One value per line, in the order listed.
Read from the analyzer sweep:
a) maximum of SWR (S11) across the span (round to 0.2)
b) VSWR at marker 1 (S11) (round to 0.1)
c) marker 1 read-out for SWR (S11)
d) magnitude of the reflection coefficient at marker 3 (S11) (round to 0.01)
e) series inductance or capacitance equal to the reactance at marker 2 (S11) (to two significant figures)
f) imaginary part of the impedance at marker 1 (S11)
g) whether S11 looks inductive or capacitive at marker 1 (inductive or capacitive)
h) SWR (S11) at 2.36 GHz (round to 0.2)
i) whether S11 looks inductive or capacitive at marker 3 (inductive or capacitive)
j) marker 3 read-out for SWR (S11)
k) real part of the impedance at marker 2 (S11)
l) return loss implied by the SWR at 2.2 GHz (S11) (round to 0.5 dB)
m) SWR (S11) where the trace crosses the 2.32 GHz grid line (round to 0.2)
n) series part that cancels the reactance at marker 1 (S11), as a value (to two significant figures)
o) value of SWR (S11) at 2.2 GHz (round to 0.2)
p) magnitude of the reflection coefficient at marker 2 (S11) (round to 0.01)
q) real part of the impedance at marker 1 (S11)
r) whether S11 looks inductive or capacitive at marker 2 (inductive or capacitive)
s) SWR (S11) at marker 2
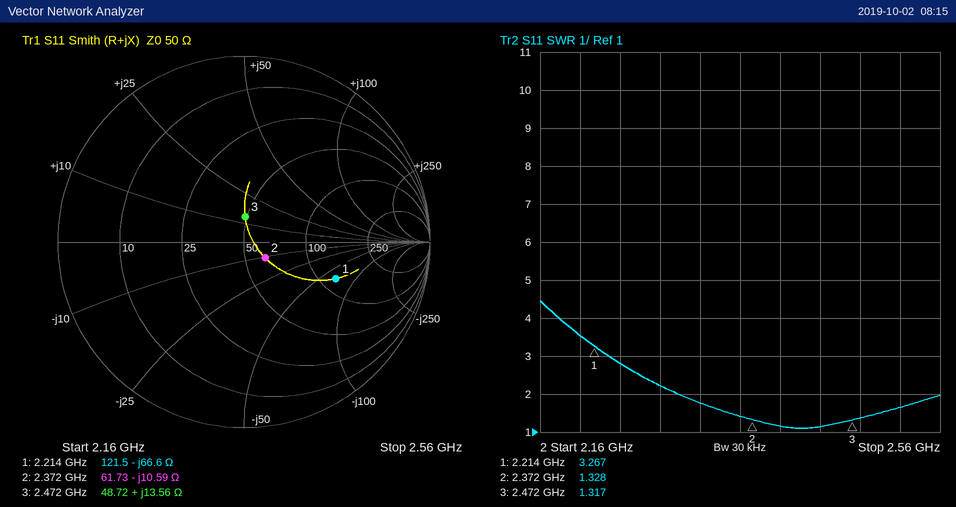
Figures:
4.4
3.3
3.267
0.14
6.3 pF
-66.6 Ω
capacitive
1.4
inductive
1.317
61.73 Ω
5.0 dB
1.8
4.8 nH
3.6
0.14
121.5 Ω
capacitive
1.328
